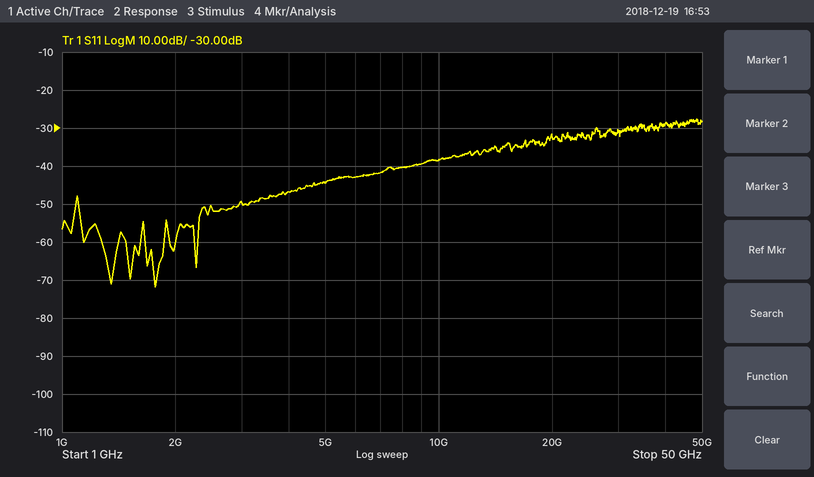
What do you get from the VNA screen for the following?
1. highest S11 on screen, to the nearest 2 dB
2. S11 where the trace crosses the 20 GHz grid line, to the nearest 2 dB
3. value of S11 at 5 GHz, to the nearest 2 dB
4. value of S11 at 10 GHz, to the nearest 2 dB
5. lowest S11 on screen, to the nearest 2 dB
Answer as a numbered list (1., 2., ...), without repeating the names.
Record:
1. -28 dB
2. -32 dB
3. -44 dB
4. -38 dB
5. -72 dB
